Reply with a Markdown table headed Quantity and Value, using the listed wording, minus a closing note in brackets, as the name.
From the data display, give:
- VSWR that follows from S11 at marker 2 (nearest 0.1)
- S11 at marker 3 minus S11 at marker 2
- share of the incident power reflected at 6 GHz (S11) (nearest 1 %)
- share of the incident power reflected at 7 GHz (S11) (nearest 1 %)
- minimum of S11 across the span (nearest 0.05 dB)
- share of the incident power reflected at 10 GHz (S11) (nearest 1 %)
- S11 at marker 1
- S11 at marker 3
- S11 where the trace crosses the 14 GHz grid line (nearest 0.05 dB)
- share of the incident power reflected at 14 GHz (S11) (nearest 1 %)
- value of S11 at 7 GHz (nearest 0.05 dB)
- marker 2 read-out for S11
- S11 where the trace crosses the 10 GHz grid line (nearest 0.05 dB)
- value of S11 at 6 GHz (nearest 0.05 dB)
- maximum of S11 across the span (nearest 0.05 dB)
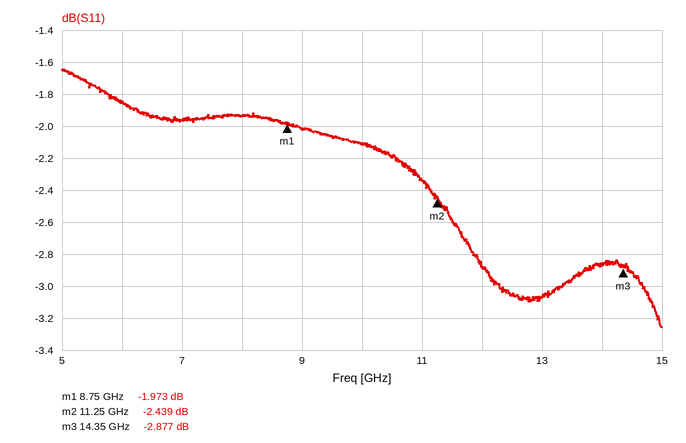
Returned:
| Quantity | Value |
|---|---|
| VSWR that follows from S11 at marker 2 | 7.2 |
| S11 at marker 3 minus S11 at marker 2 | -0.438 dB |
| share of the incident power reflected at 6 GHz (S11) | 65 % |
| share of the incident power reflected at 7 GHz (S11) | 64 % |
| minimum of S11 across the span | -3.25 dB |
| share of the incident power reflected at 10 GHz (S11) | 62 % |
| S11 at marker 1 | -1.973 dB |
| S11 at marker 3 | -2.877 dB |
| S11 where the trace crosses the 14 GHz grid line | -2.85 dB |
| share of the incident power reflected at 14 GHz (S11) | 52 % |
| value of S11 at 7 GHz | -1.95 dB |
| marker 2 read-out for S11 | -2.439 dB |
| S11 where the trace crosses the 10 GHz grid line | -2.10 dB |
| value of S11 at 6 GHz | -1.85 dB |
| maximum of S11 across the span | -1.65 dB |
